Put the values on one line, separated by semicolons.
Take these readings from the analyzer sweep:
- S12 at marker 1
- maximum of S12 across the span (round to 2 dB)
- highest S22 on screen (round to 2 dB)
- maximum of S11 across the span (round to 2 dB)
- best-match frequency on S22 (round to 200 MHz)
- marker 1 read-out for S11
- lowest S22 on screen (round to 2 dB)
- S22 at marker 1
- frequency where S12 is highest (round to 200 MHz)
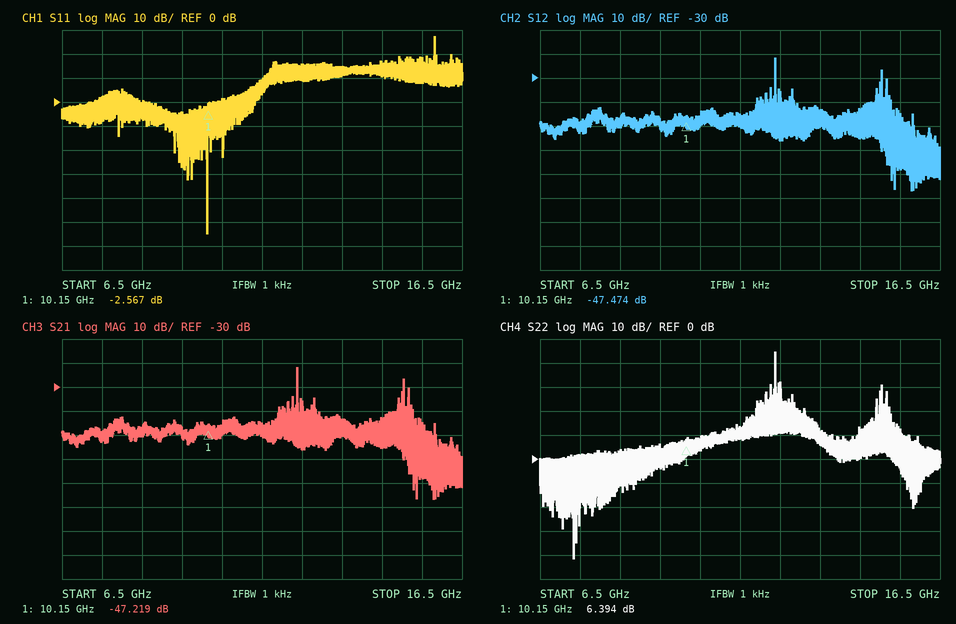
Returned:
-47.474 dB; -22 dB; 44 dB; 28 dB; 7.4 GHz; -2.567 dB; -42 dB; 6.394 dB; 12.4 GHz
